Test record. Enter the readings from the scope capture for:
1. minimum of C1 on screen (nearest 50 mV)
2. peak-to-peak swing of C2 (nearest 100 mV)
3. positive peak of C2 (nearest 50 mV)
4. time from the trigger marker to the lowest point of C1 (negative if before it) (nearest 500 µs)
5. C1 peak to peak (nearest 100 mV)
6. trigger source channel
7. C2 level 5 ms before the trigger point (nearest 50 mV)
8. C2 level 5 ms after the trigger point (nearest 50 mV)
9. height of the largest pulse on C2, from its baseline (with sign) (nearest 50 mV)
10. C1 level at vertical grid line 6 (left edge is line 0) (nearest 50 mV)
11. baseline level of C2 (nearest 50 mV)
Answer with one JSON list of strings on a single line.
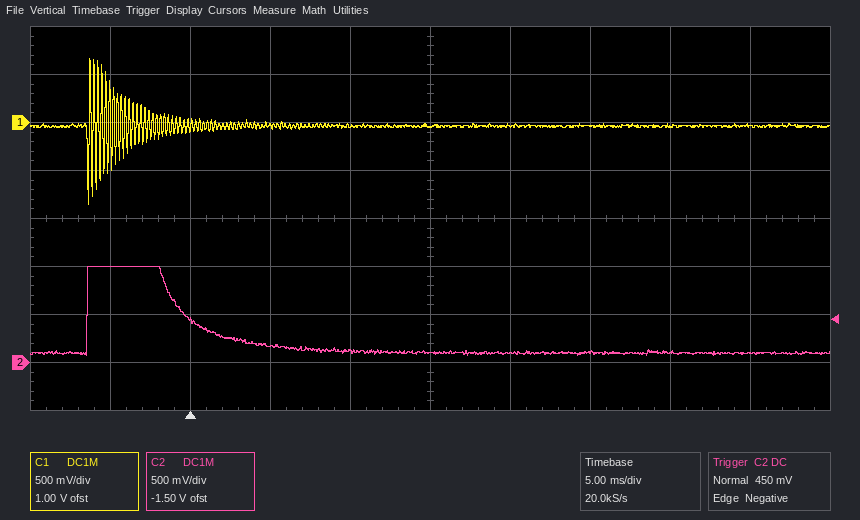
["-850 mV", "900 mV", "1.00 V", "-6.5 ms", "1.50 V", "C2", "1.00 V", "150 mV", "+900 mV", "-50 mV", "100 mV"]
